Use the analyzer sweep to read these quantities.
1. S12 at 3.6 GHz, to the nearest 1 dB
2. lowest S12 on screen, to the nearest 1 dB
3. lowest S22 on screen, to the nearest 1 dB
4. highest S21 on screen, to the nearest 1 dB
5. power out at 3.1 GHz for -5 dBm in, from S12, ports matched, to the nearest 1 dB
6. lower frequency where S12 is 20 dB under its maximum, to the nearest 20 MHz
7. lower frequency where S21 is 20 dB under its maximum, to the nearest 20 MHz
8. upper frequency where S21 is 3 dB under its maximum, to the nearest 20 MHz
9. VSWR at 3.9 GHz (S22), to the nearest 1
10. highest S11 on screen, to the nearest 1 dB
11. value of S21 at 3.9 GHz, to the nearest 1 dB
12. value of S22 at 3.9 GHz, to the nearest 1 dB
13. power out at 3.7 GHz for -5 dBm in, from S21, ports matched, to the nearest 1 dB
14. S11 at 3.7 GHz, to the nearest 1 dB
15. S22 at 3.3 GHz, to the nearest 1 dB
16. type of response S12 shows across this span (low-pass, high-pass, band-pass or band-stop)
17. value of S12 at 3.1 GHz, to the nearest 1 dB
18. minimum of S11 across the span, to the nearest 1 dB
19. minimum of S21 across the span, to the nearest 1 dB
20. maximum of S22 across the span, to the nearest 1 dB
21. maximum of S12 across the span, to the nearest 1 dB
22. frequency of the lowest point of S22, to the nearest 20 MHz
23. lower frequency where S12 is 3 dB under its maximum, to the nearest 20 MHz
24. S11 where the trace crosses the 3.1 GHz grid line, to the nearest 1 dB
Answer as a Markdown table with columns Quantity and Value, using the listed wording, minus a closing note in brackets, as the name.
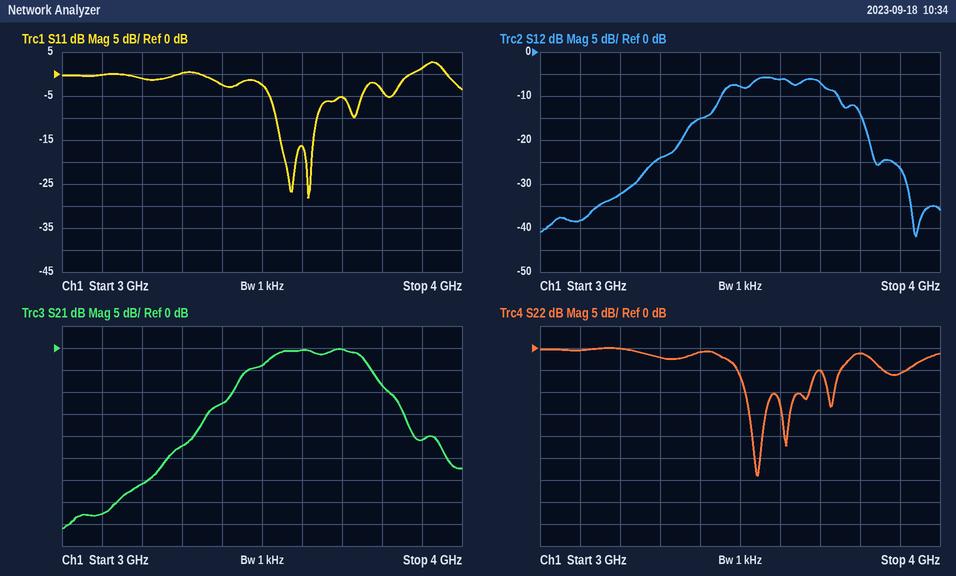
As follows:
| Quantity | Value |
|---|---|
| S12 at 3.6 GHz, to the nearest 1 dB | -6 dB |
| lowest S12 on screen, to the nearest 1 dB | -42 dB |
| lowest S22 on screen, to the nearest 1 dB | -29 dB |
| highest S21 on screen, to the nearest 1 dB | 0 dB |
| power out at 3.1 GHz for -5 dBm in, from S12, ports matched, to the nearest 1 dB | -43 dBm |
| lower frequency where S12 is 20 dB under its maximum, to the nearest 20 MHz | 3.28 GHz |
| lower frequency where S21 is 20 dB under its maximum, to the nearest 20 MHz | 3.32 GHz |
| upper frequency where S21 is 3 dB under its maximum, to the nearest 20 MHz | 3.76 GHz |
| VSWR at 3.9 GHz (S22), to the nearest 1 | 3 |
| highest S11 on screen, to the nearest 1 dB | 3 dB |
| value of S21 at 3.9 GHz, to the nearest 1 dB | -21 dB |
| value of S22 at 3.9 GHz, to the nearest 1 dB | -6 dB |
| power out at 3.7 GHz for -5 dBm in, from S21, ports matched, to the nearest 1 dB | -5 dBm |
| S11 at 3.7 GHz, to the nearest 1 dB | -5 dB |
| S22 at 3.3 GHz, to the nearest 1 dB | -2 dB |
| type of response S12 shows across this span | band-pass |
| value of S12 at 3.1 GHz, to the nearest 1 dB | -38 dB |
| minimum of S11 across the span, to the nearest 1 dB | -28 dB |
| minimum of S21 across the span, to the nearest 1 dB | -41 dB |
| maximum of S22 across the span, to the nearest 1 dB | 0 dB |
| maximum of S12 across the span, to the nearest 1 dB | -6 dB |
| frequency of the lowest point of S22, to the nearest 20 MHz | 3.54 GHz |
| lower frequency where S12 is 3 dB under its maximum, to the nearest 20 MHz | 3.46 GHz |
| S11 where the trace crosses the 3.1 GHz grid line, to the nearest 1 dB | 0 dB |
